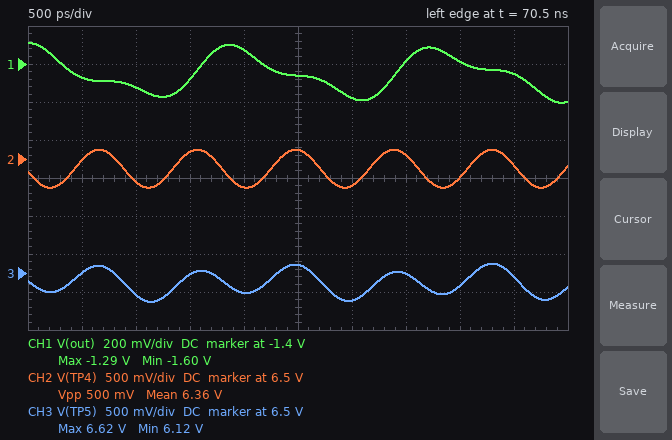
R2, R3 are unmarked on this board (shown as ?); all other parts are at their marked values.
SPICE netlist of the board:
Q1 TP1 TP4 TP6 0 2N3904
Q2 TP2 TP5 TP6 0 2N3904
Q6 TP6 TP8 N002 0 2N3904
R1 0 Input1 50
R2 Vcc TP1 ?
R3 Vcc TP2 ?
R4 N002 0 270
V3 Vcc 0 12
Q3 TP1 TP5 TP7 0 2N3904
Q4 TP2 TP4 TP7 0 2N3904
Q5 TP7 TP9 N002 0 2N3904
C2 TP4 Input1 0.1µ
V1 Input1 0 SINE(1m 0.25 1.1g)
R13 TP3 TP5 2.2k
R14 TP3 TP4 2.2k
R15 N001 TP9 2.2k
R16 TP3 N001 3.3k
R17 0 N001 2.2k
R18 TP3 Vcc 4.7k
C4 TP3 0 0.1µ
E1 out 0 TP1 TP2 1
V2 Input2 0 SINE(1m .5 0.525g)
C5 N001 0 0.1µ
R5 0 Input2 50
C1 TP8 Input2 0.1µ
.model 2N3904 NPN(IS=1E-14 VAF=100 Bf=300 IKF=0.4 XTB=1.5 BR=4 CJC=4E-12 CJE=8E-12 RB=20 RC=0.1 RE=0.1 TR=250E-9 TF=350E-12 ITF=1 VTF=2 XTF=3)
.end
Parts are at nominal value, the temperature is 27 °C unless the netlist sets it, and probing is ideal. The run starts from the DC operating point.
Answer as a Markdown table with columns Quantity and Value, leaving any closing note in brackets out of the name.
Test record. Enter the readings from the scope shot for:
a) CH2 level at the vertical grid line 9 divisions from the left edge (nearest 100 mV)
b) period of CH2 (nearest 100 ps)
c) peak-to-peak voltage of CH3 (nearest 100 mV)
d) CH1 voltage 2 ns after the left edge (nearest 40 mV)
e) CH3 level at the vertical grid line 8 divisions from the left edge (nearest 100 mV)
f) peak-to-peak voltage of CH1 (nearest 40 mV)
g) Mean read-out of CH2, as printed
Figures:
| Quantity | Value |
|---|---|
| CH2 level at the vertical grid line 9 divisions from the left edge | 6.4 V |
| period of CH2 | 900 ps |
| peak-to-peak voltage of CH3 | 500 mV |
| CH1 voltage 2 ns after the left edge | -1.32 V |
| CH3 level at the vertical grid line 8 divisions from the left edge | 6.3 V |
| peak-to-peak voltage of CH1 | 320 mV |
| Mean read-out of CH2, as printed | 6.36 V |
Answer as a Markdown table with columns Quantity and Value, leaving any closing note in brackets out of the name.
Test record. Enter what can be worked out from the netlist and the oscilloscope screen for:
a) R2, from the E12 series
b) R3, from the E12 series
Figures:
| Quantity | Value |
|---|---|
| R2, from the E12 series | 680 Ω |
| R3, from the E12 series | 220 Ω |
